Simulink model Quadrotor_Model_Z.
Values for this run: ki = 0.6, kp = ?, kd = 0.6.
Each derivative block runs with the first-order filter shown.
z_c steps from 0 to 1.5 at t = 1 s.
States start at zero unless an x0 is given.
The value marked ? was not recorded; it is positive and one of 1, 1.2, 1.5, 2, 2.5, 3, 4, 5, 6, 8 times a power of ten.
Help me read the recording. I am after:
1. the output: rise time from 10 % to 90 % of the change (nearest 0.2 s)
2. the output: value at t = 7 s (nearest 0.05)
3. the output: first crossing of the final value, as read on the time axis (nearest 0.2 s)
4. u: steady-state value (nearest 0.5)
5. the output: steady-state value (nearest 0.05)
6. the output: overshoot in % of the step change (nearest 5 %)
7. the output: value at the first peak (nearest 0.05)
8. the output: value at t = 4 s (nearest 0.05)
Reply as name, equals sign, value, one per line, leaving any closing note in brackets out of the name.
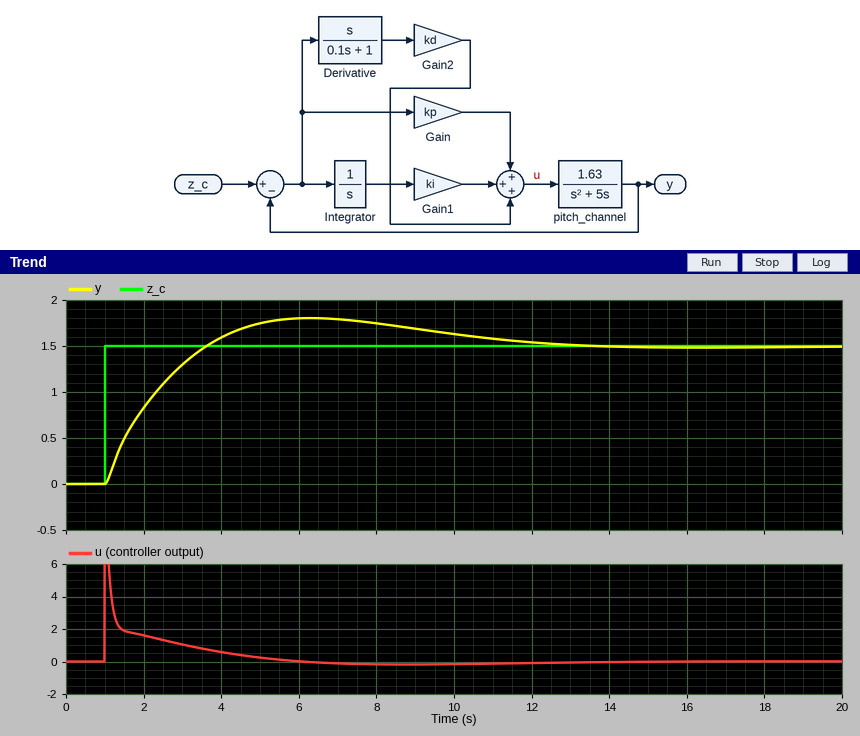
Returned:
the output: rise time from 10 % to 90 % of the change = 2.0 s
the output: value at t = 7 s = 1.80
the output: first crossing of the final value, as read on the time axis = 3.6 s
u: steady-state value = 0.0
the output: steady-state value = 1.50
the output: overshoot in % of the step change = 20 %
the output: value at the first peak = 1.80
the output: value at t = 4 s = 1.60
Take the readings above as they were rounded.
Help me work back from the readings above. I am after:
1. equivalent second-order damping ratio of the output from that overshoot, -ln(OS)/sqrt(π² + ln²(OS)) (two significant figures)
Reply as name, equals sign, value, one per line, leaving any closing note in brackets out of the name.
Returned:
equivalent second-order damping ratio of the output from that overshoot, -ln(OS)/sqrt(π² + ln²(OS)) = 0.46
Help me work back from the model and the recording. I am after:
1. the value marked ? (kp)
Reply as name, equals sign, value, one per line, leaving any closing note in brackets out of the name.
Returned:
the value marked ? = 2
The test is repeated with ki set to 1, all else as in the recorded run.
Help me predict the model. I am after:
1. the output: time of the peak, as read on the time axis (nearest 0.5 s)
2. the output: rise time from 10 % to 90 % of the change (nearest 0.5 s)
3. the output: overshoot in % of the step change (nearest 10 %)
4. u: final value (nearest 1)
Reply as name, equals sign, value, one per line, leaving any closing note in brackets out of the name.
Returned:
the output: time of the peak, as read on the time axis = 5.5 s
the output: rise time from 10 % to 90 % of the change = 1.5 s
the output: overshoot in % of the step change = 30 %
u: final value = 0
